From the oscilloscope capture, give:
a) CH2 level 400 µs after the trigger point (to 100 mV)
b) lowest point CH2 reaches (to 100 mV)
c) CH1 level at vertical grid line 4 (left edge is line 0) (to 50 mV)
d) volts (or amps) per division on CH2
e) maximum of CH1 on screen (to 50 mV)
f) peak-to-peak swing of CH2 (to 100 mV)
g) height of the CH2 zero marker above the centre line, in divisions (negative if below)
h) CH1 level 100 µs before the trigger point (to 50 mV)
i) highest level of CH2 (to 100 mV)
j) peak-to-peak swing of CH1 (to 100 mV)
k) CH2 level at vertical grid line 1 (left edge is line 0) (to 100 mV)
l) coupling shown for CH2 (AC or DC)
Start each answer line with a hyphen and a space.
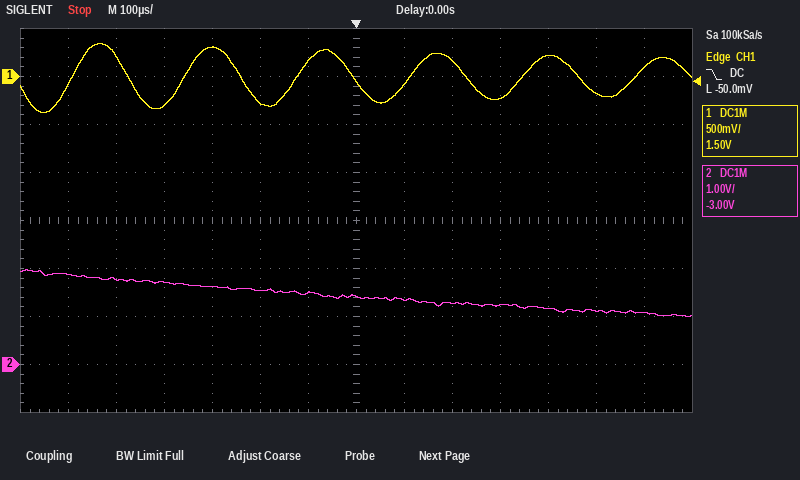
- 1.2 V
- 1.0 V
- 300 mV
- 1 V
- 350 mV
- 1.0 V
- -3.0 div
- 150 mV
- 2.0 V
- 700 mV
- 1.9 V
- DC
